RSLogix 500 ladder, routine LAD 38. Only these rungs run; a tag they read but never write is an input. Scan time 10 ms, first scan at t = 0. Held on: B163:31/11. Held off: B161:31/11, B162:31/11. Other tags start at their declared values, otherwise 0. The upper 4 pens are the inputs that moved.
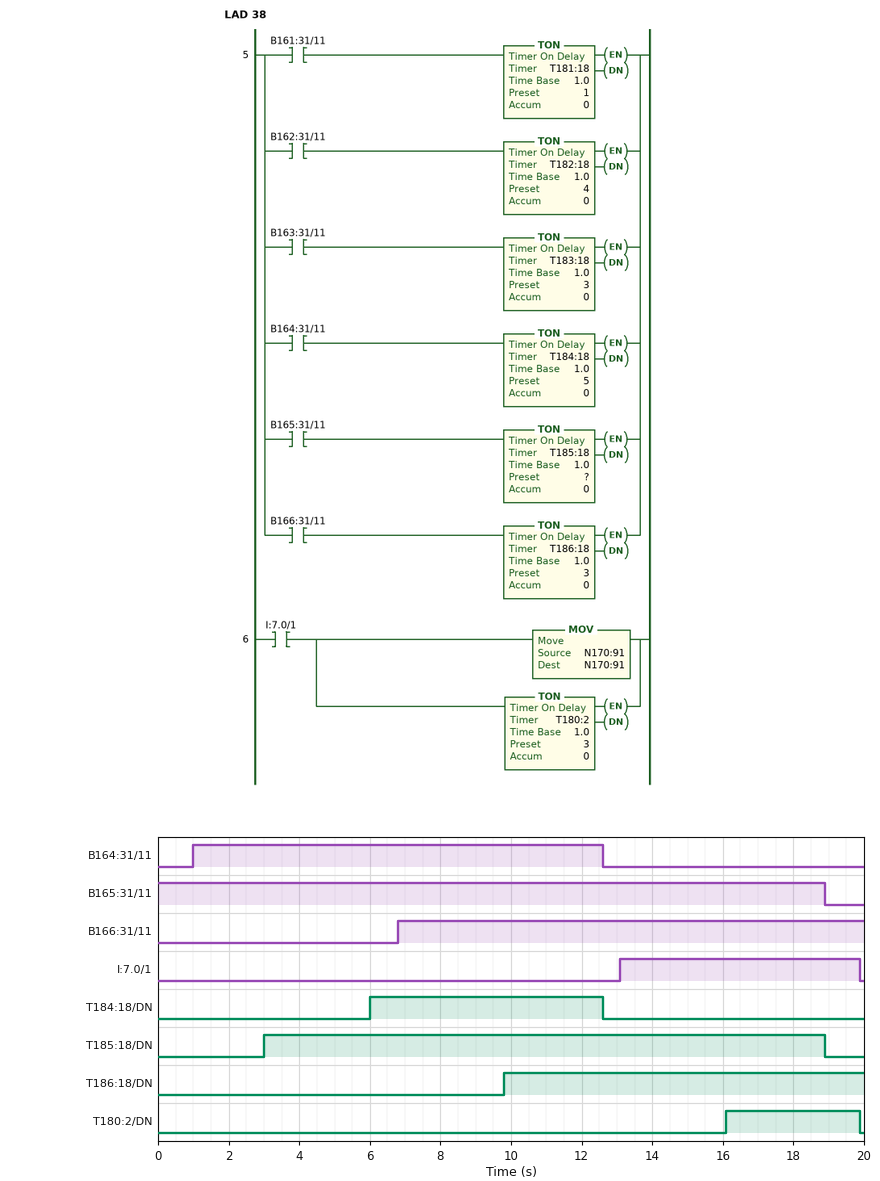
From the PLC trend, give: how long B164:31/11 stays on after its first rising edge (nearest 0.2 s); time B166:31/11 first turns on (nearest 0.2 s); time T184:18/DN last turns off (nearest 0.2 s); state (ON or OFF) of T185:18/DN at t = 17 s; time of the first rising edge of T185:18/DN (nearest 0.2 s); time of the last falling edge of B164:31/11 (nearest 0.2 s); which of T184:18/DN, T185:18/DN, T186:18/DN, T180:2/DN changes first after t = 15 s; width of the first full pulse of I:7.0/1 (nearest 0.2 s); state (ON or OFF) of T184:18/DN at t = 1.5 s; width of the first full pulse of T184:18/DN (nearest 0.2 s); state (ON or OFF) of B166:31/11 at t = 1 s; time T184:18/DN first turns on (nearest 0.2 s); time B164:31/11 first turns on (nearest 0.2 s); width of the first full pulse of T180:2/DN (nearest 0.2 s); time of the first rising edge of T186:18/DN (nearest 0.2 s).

11.6 s
6.8 s
12.6 s
ON
3.0 s
12.6 s
T180:2/DN
6.8 s
OFF
6.6 s
OFF
6.0 s
1.0 s
3.8 s
9.8 s
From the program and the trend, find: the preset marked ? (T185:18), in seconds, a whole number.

3 s
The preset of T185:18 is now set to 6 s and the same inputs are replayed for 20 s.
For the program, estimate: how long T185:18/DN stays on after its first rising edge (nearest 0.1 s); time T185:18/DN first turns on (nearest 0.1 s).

12.9 s
6.0 s
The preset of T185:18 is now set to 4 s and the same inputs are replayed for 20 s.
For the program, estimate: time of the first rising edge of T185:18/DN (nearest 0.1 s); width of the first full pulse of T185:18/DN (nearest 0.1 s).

4.0 s
14.9 s
